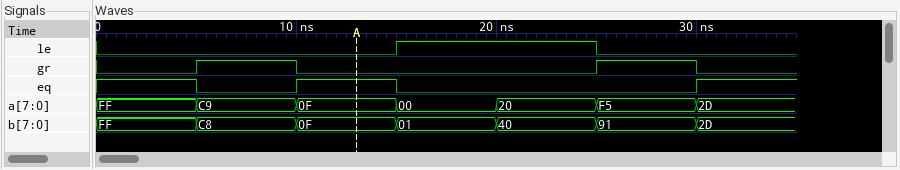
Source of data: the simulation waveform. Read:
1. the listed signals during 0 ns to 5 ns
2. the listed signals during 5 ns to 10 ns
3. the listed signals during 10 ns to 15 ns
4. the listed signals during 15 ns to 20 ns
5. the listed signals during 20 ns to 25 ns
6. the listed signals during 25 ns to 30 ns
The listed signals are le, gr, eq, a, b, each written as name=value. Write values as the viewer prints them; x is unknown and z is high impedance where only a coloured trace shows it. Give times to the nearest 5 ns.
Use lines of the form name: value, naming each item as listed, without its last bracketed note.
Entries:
the listed signals during 0 ns to 5 ns: le=0, gr=0, eq=1, a=FF, b=FF
the listed signals during 5 ns to 10 ns: le=0, gr=1, eq=0, a=C9, b=C8
the listed signals during 10 ns to 15 ns: le=0, gr=0, eq=1, a=0F, b=0F
the listed signals during 15 ns to 20 ns: le=1, gr=0, eq=0, a=00, b=01
the listed signals during 20 ns to 25 ns: le=1, gr=0, eq=0, a=20, b=40
the listed signals during 25 ns to 30 ns: le=0, gr=1, eq=0, a=F5, b=91
